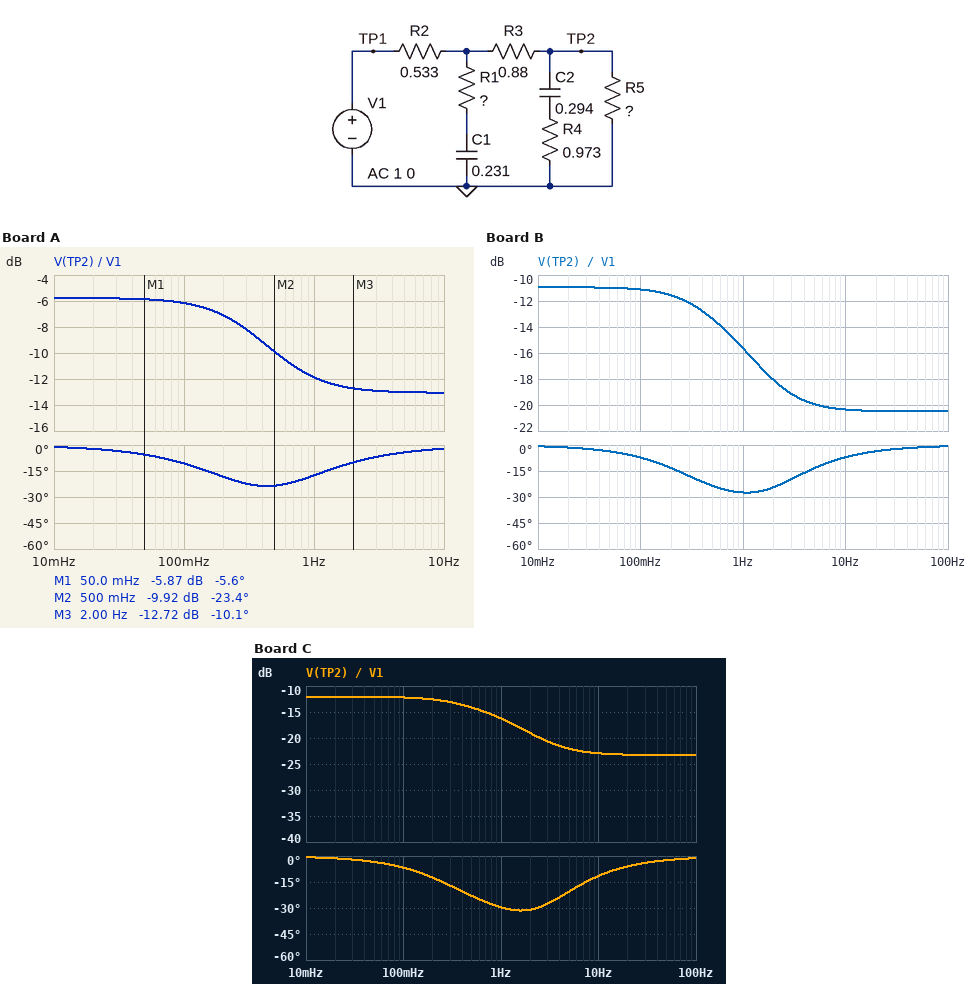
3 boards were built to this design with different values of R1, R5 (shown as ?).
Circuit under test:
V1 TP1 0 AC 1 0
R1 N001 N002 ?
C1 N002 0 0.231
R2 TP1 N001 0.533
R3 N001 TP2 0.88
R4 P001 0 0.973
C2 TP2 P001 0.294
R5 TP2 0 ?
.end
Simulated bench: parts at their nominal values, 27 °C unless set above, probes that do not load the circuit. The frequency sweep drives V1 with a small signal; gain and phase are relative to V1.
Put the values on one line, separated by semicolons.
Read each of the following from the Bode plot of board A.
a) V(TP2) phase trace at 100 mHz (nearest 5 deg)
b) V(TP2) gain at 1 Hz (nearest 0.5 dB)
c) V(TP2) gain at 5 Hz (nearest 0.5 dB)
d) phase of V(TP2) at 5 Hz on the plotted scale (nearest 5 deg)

-10 deg; -12.0 dB; -13.0 dB; -5 deg
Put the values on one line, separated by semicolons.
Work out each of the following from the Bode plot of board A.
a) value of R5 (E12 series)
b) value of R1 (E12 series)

1.5 Ω; 1.2 Ω
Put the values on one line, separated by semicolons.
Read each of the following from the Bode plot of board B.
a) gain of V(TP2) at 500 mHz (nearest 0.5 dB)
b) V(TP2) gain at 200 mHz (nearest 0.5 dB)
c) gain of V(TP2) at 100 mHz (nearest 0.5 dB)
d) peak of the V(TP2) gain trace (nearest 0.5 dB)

-13.5 dB; -11.5 dB; -11.0 dB; -11.0 dB
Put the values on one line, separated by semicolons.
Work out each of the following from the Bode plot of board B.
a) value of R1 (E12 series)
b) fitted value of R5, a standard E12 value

0.33 Ω; 0.56 Ω
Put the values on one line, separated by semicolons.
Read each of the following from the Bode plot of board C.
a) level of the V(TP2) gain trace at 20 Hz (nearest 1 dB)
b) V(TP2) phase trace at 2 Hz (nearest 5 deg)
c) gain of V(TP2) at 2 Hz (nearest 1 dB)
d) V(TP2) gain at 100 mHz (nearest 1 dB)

-23 dB; -30 deg; -19 dB; -12 dB
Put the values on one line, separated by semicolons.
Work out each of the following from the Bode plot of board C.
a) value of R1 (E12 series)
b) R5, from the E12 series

0.22 Ω; 0.47 Ω
